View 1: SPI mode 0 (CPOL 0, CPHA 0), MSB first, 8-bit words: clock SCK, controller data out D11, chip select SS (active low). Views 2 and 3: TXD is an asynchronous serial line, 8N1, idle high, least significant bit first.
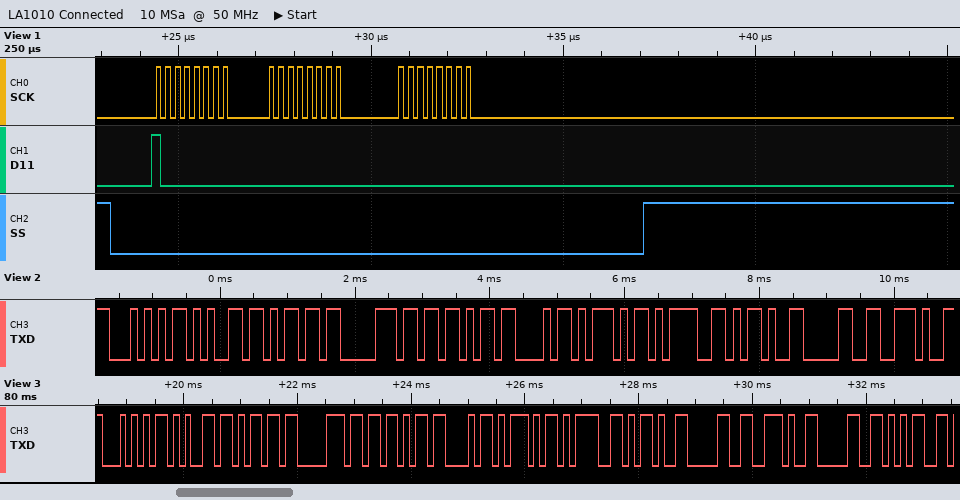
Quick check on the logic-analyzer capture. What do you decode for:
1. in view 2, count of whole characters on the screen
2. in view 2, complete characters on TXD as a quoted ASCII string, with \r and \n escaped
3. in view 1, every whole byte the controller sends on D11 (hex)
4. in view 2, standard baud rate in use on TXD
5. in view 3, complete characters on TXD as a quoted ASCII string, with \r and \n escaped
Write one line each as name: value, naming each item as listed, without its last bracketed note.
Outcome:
in view 2, count of whole characters on the screen: 11
in view 2, complete characters on TXD as a quoted ASCII string, with \r and \n escaped: "Temp[C]=-0."
in view 1, every whole byte the controller sends on D11: 0x80 0x00 0x00
in view 2, standard baud rate in use on TXD: 9600 baud
in view 3, complete characters on TXD as a quoted ASCII string, with \r and \n escaped: "Temp[C]=-0.05"
